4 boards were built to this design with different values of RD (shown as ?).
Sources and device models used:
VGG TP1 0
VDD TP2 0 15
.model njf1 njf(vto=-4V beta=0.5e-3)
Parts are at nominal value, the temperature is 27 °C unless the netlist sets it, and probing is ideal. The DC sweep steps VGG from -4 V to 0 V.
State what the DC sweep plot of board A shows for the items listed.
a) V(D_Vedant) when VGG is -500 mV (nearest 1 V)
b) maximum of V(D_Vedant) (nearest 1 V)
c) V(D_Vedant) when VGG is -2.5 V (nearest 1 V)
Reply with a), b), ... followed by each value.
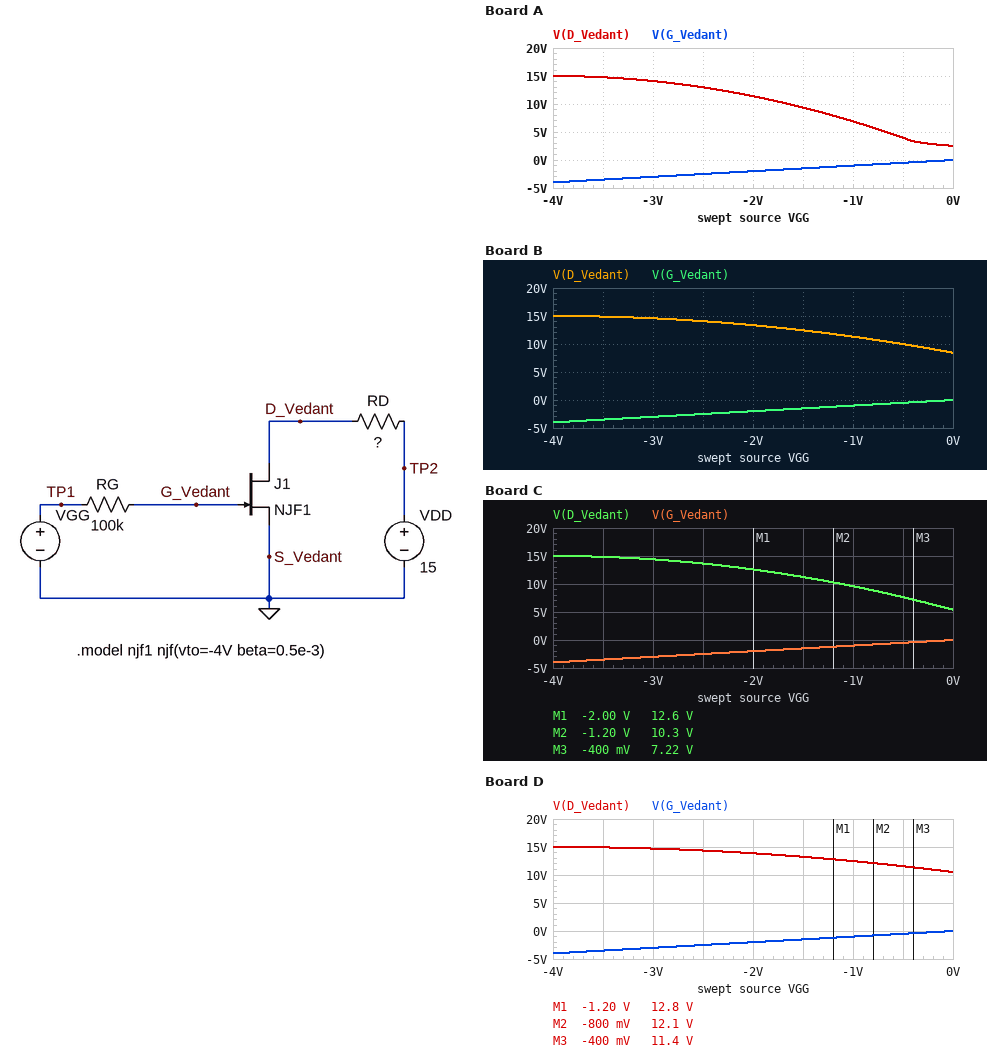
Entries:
a) 4 V
b) 15 V
c) 13 V
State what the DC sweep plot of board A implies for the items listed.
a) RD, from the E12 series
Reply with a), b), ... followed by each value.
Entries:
a) 1.8 kΩ
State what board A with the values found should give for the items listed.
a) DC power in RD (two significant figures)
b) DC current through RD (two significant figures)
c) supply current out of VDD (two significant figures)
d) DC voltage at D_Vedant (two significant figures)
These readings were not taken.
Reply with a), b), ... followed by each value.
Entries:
a) 86 mW
b) 6.9 mA
c) 6.9 mA
d) 2.5 V
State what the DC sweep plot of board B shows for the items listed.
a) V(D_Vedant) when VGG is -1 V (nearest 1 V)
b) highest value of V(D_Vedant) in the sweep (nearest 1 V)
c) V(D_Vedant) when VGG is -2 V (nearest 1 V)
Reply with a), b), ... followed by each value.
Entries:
a) 11 V
b) 15 V
c) 13 V
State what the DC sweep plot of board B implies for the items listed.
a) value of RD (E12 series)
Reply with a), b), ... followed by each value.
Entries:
a) 820 Ω
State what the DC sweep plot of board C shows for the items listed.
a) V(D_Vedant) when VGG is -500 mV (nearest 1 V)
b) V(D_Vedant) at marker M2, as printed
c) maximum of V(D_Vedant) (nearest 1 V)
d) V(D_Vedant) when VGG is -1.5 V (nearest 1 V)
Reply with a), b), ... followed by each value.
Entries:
a) 8 V
b) 10.3 V
c) 15 V
d) 11 V
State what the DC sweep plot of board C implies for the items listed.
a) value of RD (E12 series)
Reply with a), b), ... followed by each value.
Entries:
a) 1.2 kΩ
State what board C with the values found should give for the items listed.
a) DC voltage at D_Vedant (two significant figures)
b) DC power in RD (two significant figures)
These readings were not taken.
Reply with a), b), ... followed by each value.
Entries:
a) 5.4 V
b) 77 mW
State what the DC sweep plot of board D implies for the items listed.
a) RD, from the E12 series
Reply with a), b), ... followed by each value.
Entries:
a) 560 Ω
